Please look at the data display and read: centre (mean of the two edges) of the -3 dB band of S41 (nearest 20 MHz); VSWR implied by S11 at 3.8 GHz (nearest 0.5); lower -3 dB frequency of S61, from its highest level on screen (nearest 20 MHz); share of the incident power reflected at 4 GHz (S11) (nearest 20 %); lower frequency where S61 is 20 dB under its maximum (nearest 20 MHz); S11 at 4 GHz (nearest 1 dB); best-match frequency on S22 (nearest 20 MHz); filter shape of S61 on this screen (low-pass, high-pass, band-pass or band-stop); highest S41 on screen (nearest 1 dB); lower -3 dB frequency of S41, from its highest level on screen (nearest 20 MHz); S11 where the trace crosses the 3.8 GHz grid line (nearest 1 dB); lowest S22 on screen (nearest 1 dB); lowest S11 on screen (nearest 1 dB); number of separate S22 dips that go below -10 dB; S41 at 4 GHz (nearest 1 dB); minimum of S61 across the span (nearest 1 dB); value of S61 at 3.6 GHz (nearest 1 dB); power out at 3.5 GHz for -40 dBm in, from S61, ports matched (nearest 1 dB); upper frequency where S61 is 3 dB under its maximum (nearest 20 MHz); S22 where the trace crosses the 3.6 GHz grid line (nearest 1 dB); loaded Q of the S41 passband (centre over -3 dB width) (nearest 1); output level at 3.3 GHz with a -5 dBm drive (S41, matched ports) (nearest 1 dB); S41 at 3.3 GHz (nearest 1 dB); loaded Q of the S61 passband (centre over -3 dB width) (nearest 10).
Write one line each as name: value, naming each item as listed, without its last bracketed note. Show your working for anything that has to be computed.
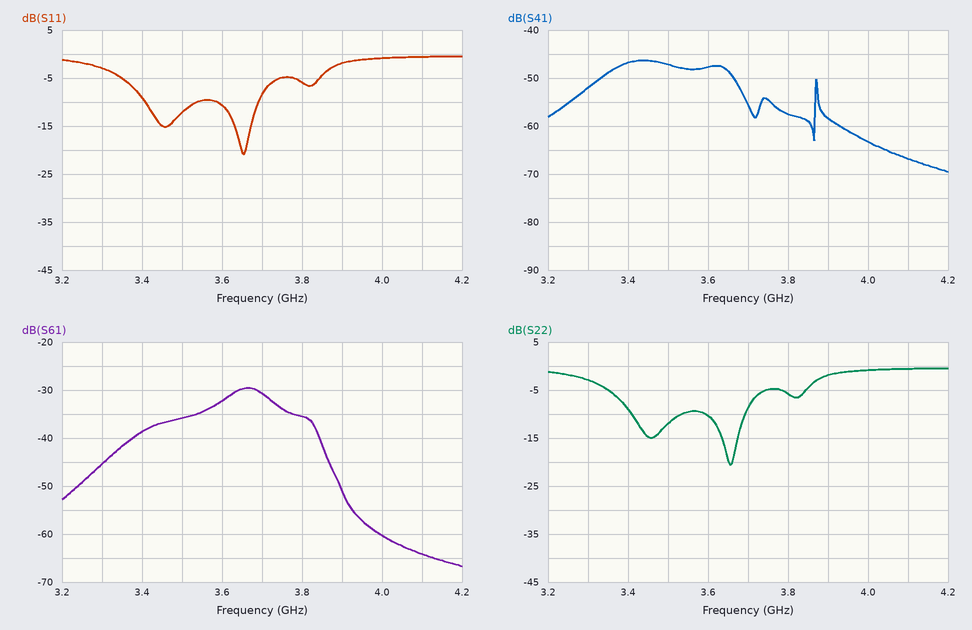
centre (mean of the two edges) of the -3 dB band of S41: 3.50 GHz
VSWR implied by S11 at 3.8 GHz: |Γ| = 10^(-6/20) = 0.5012; VSWR = (1 + 0.5012)/(1 − 0.5012) ≈ 3.0
lower -3 dB frequency of S61, from its highest level on screen: 3.60 GHz
share of the incident power reflected at 4 GHz (S11): 10^(-1/10) ≈ 79.4 %, so 80 % to the nearest 20 %
lower frequency where S61 is 20 dB under its maximum: 3.24 GHz
S11 at 4 GHz: -1 dB
best-match frequency on S22: 3.66 GHz
filter shape of S61 on this screen: band-pass
highest S41 on screen: -46 dB
lower -3 dB frequency of S41, from its highest level on screen: 3.34 GHz
S11 where the trace crosses the 3.8 GHz grid line: -6 dB
lowest S22 on screen: -21 dB
lowest S11 on screen: -21 dB
number of separate S22 dips that go below -10 dB: 2
S41 at 4 GHz: -63 dB
minimum of S61 across the span: -67 dB
value of S61 at 3.6 GHz: -32 dB
power out at 3.5 GHz for -40 dBm in, from S61, ports matched: -40 dBm + (-36 dB) = -76 dBm
upper frequency where S61 is 3 dB under its maximum: 3.72 GHz
S22 where the trace crosses the 3.6 GHz grid line: -10 dB
loaded Q of the S41 passband (centre over -3 dB width): 3.5 GHz / 320 MHz ≈ 11
output level at 3.3 GHz with a -5 dBm drive (S41, matched ports): -5 dBm + (-52 dB) = -57 dBm
S41 at 3.3 GHz: -52 dB
loaded Q of the S61 passband (centre over -3 dB width): 3.66 GHz / 120 MHz ≈ 30
